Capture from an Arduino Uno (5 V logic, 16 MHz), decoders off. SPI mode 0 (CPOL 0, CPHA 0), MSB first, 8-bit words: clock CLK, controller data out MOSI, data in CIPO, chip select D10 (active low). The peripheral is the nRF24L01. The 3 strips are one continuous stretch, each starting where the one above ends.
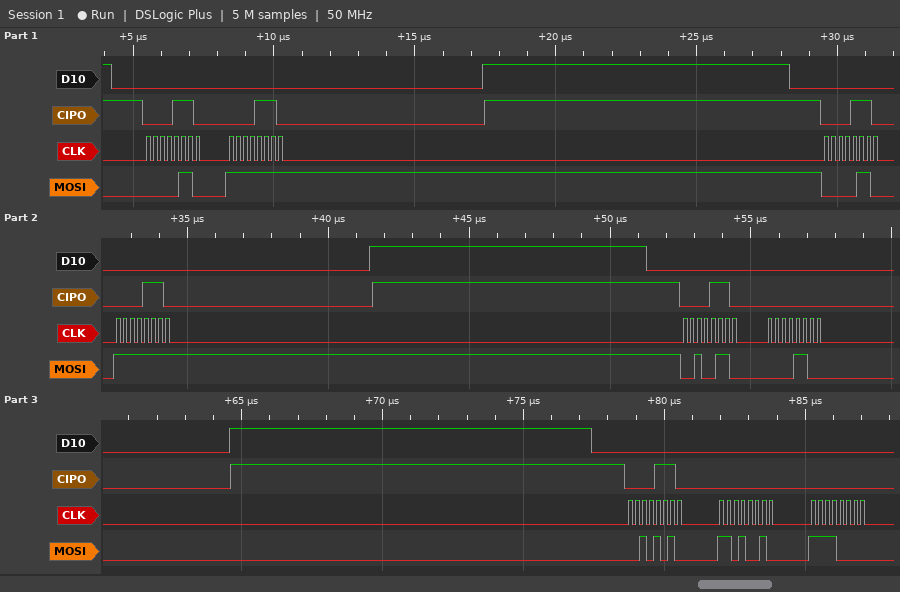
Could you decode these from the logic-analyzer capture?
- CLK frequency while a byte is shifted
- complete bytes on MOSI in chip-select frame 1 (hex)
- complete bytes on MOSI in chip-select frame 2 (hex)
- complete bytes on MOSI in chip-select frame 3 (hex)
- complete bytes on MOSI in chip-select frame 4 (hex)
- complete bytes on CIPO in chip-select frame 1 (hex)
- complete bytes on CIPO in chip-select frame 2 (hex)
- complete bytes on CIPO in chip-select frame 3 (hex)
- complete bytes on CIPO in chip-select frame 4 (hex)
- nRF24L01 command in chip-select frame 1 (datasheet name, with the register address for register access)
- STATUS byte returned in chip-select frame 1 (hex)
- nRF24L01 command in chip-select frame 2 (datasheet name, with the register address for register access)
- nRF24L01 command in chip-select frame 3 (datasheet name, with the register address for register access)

4 MHz
06 FF
06 FF
26 0C
2A D2 F0
0E 0E
0E 0E
0E 00
0E 00 00
R_REGISTER 0x06
0x0E
R_REGISTER 0x06
W_REGISTER 0x06
